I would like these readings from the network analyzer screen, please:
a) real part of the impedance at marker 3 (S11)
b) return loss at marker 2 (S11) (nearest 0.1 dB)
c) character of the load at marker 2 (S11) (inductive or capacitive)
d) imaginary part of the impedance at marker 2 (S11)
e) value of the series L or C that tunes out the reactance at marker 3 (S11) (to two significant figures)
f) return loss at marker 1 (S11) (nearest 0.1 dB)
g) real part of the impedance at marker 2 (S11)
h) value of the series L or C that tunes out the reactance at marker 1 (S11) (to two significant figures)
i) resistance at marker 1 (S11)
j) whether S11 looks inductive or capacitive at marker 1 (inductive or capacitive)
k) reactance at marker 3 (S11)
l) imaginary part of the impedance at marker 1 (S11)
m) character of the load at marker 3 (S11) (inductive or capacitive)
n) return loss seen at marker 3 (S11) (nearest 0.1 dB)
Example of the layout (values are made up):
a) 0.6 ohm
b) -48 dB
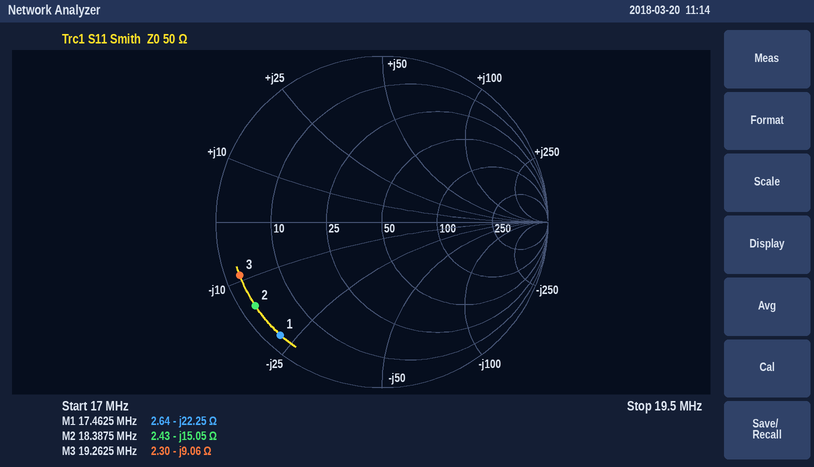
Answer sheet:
a) 2.30 Ω
b) 0.8 dB
c) capacitive
d) -15.05 Ω
e) 75 nH
f) 0.8 dB
g) 2.43 Ω
h) 200 nH
i) 2.64 Ω
j) capacitive
k) -9.06 Ω
l) -22.25 Ω
m) capacitive
n) 0.8 dB
